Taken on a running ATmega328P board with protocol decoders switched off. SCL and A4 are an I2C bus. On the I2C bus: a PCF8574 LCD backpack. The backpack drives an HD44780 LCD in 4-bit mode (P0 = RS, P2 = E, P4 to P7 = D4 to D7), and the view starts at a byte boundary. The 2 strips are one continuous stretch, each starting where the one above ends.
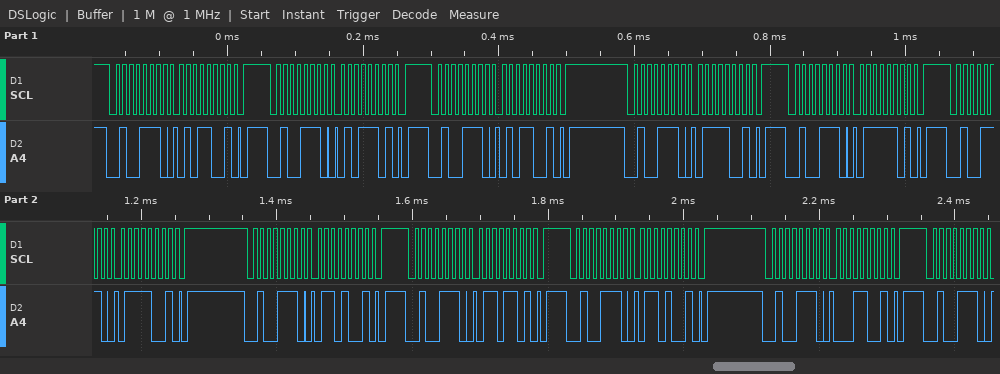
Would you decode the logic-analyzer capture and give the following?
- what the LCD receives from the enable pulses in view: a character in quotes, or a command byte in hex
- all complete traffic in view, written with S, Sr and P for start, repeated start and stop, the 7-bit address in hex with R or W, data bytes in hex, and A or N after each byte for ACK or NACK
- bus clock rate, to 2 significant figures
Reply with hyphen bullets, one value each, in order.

- 'W'
- S 27W A 59 A P S 27W A 5D A P S 27W A 59 A P S 27W A 79 A P S 27W A 7D A P S 27W A 79 A P S 27W A 69 A P S 27W A 6D A P S 27W A 69 A P S 27W A 19 A P S 27W A
- 100 kHz
